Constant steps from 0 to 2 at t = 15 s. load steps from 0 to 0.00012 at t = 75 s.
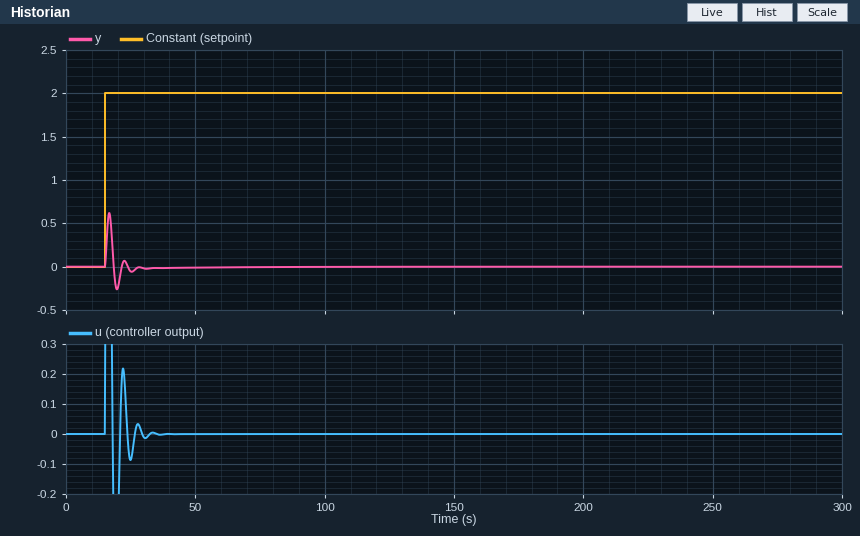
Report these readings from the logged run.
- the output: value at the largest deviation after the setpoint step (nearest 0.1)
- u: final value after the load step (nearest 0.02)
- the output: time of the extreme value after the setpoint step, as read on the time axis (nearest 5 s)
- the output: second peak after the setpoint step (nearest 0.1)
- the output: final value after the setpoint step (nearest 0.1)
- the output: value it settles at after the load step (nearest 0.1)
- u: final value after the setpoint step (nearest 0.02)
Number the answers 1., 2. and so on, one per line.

1. 0.6
2. 0.00
3. 15 s
4. 0.1
5. 0.0
6. 0.0
7. 0.00
